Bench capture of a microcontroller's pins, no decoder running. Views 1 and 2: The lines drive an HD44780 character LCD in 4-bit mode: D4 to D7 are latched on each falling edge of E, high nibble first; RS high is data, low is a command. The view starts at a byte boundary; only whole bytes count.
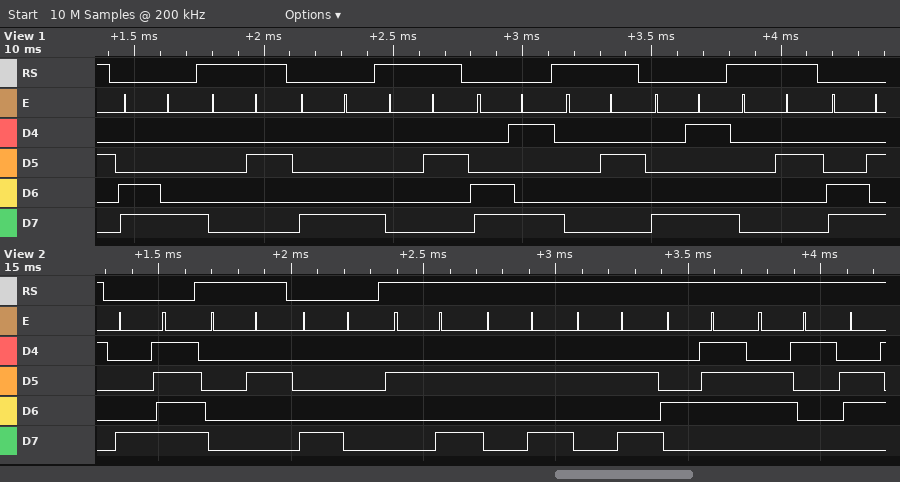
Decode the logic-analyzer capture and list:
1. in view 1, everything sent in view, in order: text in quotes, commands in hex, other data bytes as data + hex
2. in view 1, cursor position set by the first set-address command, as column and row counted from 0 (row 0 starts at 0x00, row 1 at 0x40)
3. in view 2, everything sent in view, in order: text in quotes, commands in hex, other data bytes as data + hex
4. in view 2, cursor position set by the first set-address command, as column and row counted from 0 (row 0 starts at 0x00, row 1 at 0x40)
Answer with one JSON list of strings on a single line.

["0xC8 data 02 0x88 data 02 0xC9 data 02 0x89 data 02 0xCA", "column 8, row 1", "0x8F data 02 0x80 \"***Ga\"", "column 15, row 0"]
